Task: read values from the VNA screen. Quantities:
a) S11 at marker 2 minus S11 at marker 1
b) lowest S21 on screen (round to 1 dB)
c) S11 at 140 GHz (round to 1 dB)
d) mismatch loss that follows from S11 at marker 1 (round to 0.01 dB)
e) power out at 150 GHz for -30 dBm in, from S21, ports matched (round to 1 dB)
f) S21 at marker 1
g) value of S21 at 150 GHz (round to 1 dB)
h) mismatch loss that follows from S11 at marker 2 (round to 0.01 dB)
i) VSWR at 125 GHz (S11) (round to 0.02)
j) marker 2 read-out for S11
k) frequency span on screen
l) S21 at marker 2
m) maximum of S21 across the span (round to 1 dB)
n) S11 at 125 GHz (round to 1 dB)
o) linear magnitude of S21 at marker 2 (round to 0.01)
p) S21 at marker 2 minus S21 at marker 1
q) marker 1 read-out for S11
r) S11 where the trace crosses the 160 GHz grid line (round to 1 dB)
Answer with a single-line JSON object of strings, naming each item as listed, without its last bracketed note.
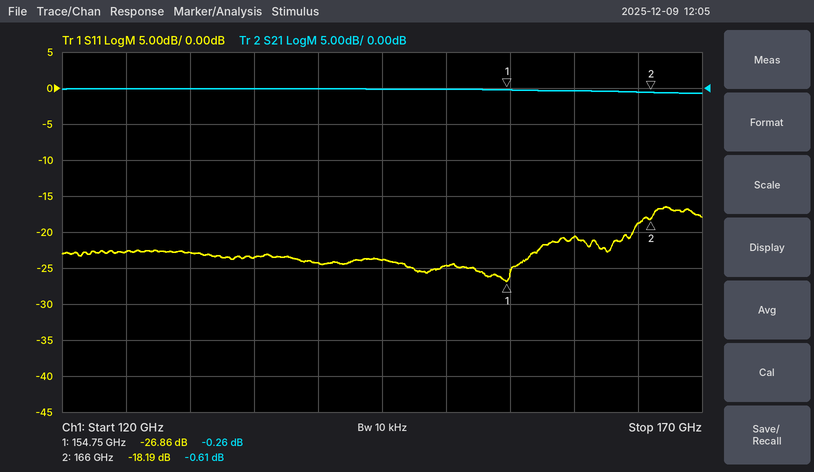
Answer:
{"S11 at marker 2 minus S11 at marker 1": "8.67 dB", "lowest S21 on screen": "-1 dB", "S11 at 140 GHz": "-24 dB", "mismatch loss that follows from S11 at marker 1": "0.01 dB", "power out at 150 GHz for -30 dBm in, from S21, ports matched": "-30 dBm", "S21 at marker 1": "-0.26 dB", "value of S21 at 150 GHz": "0 dB", "mismatch loss that follows from S11 at marker 2": "0.07 dB", "VSWR at 125 GHz (S11)": "1.16", "marker 2 read-out for S11": "-18.19 dB", "frequency span on screen": "50 GHz", "S21 at marker 2": "-0.61 dB", "maximum of S21 across the span": "0 dB", "S11 at 125 GHz": "-23 dB", "linear magnitude of S21 at marker 2": "0.93", "S21 at marker 2 minus S21 at marker 1": "-0.35 dB", "marker 1 read-out for S11": "-26.86 dB", "S11 where the trace crosses the 160 GHz grid line": "-21 dB"}
